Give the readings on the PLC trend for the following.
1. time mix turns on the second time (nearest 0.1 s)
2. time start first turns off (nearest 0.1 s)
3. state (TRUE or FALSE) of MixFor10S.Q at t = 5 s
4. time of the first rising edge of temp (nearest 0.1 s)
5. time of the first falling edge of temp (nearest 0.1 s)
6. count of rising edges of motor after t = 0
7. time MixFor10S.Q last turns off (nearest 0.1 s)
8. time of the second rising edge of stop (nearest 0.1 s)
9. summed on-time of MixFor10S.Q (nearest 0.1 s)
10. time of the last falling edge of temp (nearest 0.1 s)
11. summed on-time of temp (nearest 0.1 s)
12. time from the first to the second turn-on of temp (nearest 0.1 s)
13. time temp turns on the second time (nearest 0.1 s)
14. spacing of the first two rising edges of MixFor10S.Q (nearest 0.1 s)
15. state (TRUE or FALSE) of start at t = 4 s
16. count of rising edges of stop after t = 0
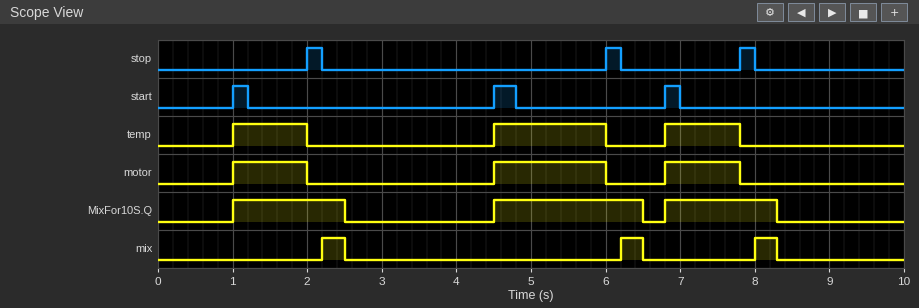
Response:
6.2 s
1.2 s
TRUE
1.0 s
2.0 s
3
8.3 s
6.0 s
5.0 s
7.8 s
3.5 s
3.5 s
4.5 s
3.5 s
FALSE
3
